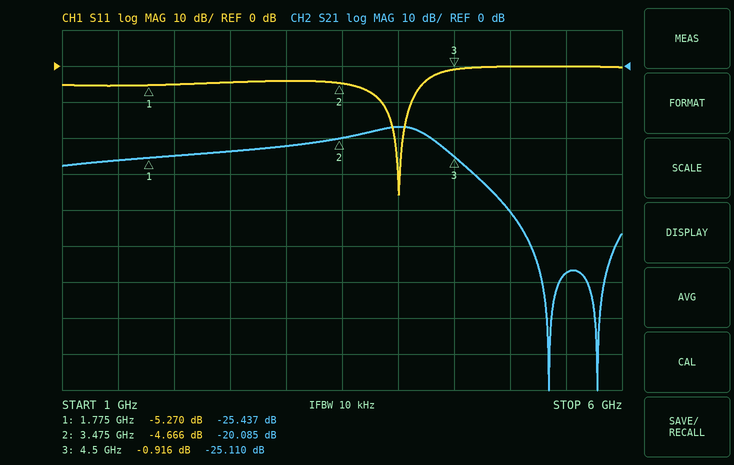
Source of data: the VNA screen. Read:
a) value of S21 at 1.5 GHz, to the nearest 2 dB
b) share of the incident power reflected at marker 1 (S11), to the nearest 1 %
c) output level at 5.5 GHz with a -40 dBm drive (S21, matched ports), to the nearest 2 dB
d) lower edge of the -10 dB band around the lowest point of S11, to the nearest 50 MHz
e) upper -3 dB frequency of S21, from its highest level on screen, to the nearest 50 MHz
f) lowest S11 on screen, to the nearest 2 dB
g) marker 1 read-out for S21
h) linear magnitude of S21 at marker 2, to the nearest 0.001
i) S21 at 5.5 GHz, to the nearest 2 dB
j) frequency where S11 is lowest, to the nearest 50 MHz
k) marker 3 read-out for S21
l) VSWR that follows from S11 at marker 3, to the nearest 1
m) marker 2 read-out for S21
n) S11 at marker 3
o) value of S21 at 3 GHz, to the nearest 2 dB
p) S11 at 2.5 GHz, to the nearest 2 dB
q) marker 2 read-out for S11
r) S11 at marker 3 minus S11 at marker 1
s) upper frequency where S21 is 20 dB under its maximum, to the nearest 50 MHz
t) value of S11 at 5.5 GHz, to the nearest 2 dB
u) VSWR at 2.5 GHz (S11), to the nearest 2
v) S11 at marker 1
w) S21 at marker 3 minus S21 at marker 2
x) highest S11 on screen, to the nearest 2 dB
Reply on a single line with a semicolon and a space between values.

-26 dB; 30 %; -98 dBm; 3.85 GHz; 4.30 GHz; -36 dB; -25.437 dB; 0.099; -58 dB; 4.00 GHz; -25.110 dB; 19; -20.085 dB; -0.916 dB; -22 dB; -4 dB; -4.666 dB; 4.354 dB; 4.90 GHz; 0 dB; 4; -5.270 dB; -5.025 dB; 0 dB
